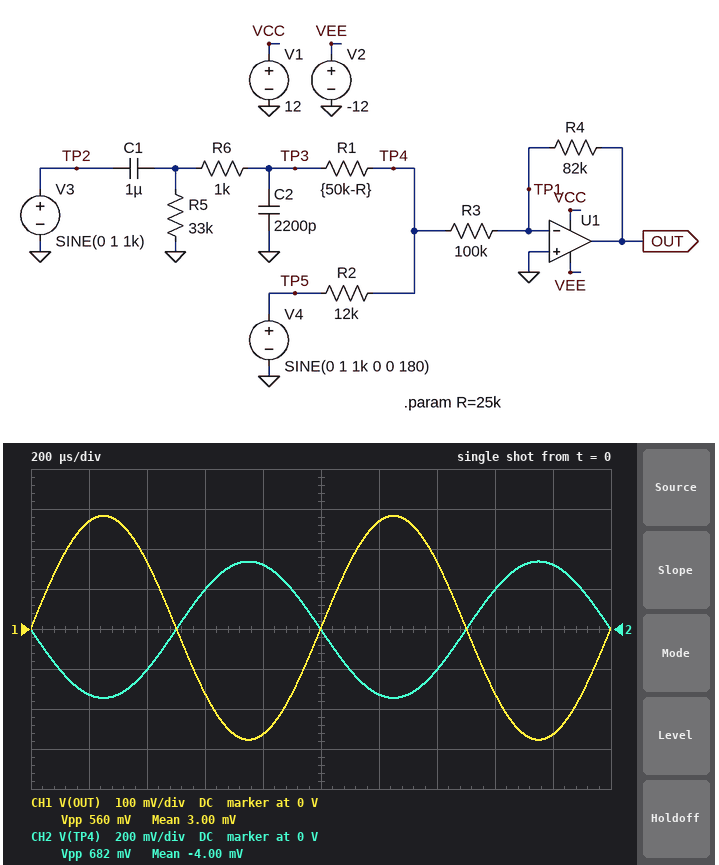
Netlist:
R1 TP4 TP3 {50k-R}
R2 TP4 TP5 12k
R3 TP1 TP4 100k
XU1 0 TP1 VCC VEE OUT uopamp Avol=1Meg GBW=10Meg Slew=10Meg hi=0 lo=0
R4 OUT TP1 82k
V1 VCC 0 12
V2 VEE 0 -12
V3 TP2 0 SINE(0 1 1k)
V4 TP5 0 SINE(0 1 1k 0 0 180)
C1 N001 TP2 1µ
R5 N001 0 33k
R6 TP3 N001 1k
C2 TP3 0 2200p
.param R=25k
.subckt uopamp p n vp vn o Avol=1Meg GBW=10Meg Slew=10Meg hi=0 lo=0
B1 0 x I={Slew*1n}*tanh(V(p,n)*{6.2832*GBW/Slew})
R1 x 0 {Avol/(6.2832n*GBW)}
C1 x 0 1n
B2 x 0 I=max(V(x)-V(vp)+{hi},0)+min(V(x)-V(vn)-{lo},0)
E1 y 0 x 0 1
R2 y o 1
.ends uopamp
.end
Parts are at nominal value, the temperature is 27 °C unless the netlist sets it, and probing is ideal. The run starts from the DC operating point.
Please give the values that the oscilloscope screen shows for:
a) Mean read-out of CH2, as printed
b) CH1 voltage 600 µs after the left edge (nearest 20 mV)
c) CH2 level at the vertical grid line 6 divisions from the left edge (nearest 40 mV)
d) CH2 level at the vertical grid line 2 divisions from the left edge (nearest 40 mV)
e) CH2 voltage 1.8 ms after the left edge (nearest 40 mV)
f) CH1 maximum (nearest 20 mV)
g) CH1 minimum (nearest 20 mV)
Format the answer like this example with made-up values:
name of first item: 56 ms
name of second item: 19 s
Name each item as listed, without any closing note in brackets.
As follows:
Mean read-out of CH2, as printed: -4.00 mV
CH1 voltage 600 µs after the left edge: -160 mV
CH2 level at the vertical grid line 6 divisions from the left edge: -320 mV
CH2 level at the vertical grid line 2 divisions from the left edge: -200 mV
CH2 voltage 1.8 ms after the left edge: 320 mV
CH1 maximum: 280 mV
CH1 minimum: -280 mV
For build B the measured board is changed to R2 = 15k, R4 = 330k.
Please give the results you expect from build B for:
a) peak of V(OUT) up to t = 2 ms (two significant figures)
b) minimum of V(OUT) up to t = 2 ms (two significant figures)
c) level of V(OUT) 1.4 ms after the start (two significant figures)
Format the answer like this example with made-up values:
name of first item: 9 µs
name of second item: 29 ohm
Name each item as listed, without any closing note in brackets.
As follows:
peak of V(OUT) up to t = 2 ms: 820 mV
minimum of V(OUT) up to t = 2 ms: -800 mV
level of V(OUT) 1.4 ms after the start: 490 mV
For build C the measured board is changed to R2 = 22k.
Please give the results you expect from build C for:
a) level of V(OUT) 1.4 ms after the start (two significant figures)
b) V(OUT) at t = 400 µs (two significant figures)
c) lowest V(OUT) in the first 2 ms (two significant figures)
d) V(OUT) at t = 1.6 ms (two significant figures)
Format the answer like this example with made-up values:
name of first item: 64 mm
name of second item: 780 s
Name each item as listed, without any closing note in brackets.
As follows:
level of V(OUT) 1.4 ms after the start: 39 mV
V(OUT) at t = 400 µs: 40 mV
lowest V(OUT) in the first 2 ms: -58 mV
V(OUT) at t = 1.6 ms: -33 mV
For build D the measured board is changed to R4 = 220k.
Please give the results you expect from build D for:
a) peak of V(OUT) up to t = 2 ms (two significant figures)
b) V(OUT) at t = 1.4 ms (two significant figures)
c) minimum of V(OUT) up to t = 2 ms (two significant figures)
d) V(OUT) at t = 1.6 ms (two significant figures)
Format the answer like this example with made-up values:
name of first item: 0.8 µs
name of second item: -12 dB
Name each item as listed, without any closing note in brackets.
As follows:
peak of V(OUT) up to t = 2 ms: 760 mV
V(OUT) at t = 1.4 ms: 450 mV
minimum of V(OUT) up to t = 2 ms: -740 mV
V(OUT) at t = 1.6 ms: -430 mV
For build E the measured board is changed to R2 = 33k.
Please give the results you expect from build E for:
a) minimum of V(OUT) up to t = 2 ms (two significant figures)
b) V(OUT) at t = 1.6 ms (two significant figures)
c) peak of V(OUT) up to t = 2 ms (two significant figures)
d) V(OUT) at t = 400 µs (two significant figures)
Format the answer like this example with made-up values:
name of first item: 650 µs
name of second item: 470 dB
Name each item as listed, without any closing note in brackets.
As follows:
minimum of V(OUT) up to t = 2 ms: -80 mV
V(OUT) at t = 1.6 ms: 52 mV
peak of V(OUT) up to t = 2 ms: 88 mV
V(OUT) at t = 400 µs: -46 mV
